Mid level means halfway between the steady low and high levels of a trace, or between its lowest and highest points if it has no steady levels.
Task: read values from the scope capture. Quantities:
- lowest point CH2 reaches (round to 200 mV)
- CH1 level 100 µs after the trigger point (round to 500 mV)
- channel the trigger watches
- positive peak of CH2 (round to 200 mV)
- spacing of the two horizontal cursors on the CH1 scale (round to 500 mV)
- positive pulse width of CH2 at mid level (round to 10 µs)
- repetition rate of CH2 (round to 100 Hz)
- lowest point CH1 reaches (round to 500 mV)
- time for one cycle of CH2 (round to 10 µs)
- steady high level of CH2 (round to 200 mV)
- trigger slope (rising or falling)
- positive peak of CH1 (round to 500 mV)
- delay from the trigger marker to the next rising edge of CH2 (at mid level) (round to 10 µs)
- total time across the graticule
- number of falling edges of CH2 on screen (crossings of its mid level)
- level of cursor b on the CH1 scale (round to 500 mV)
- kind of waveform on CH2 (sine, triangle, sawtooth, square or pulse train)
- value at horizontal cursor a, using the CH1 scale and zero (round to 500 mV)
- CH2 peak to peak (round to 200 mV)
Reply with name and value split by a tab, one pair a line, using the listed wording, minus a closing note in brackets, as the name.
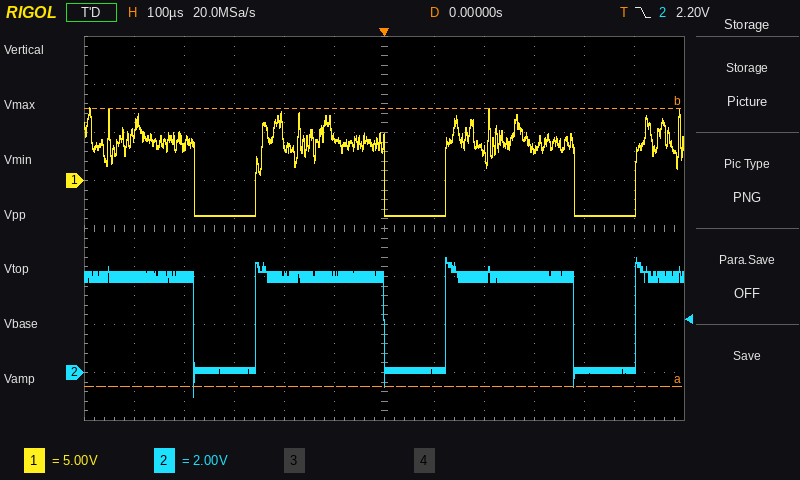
lowest point CH2 reaches	-1.0 V
CH1 level 100 µs after the trigger point	-3.5 V
channel the trigger watches	CH2
positive peak of CH2	4.8 V
spacing of the two horizontal cursors on the CH1 scale	29.0 V
positive pulse width of CH2 at mid level	260 µs
repetition rate of CH2	2.6 kHz
lowest point CH1 reaches	-3.5 V
time for one cycle of CH2	380 µs
steady high level of CH2	4.0 V
trigger slope	falling
positive peak of CH1	7.5 V
delay from the trigger marker to the next rising edge of CH2 (at mid level)	120 µs
total time across the graticule	1.2 ms
number of falling edges of CH2 on screen	3
level of cursor b on the CH1 scale	7.5 V
kind of waveform on CH2	pulse train
value at horizontal cursor a, using the CH1 scale and zero	-21.5 V
CH2 peak to peak	5.8 V
